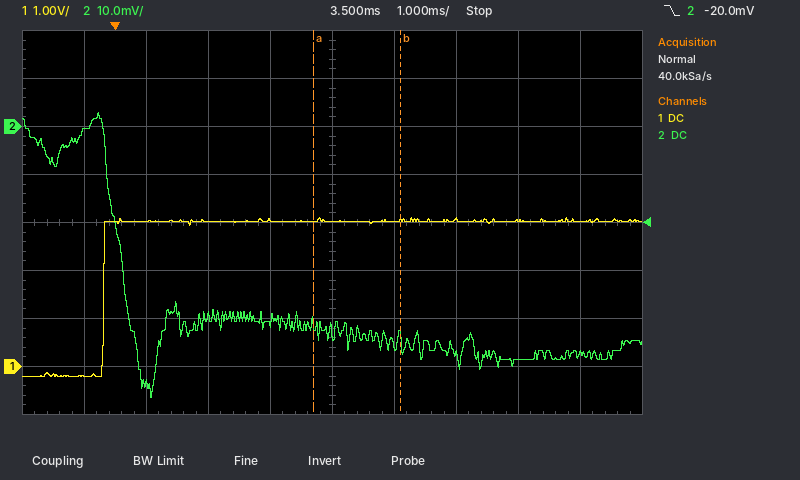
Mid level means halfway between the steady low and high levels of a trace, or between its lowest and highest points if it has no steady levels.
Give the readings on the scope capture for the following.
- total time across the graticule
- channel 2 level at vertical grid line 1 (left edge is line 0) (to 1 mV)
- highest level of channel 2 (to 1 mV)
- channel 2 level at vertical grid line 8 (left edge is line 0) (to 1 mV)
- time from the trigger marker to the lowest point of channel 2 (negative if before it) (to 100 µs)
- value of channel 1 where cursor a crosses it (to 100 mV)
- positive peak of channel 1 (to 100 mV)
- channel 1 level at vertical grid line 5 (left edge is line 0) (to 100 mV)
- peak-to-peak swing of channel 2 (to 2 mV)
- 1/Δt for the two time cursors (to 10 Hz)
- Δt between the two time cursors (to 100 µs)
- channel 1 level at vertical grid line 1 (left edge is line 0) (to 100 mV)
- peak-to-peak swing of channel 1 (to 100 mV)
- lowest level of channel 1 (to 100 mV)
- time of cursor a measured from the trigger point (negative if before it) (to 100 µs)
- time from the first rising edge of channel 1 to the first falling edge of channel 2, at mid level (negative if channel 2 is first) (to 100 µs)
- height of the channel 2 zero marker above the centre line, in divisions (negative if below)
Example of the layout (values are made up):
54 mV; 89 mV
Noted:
10 ms; -1 mV; 3 mV; -49 mV; +600 µs; 3.0 V; 3.1 V; 3.0 V; 60 mV; 710 Hz; 1.4 ms; -200 mV; 3.3 V; -200 mV; +3.2 ms; +300 µs; +2.0 div
